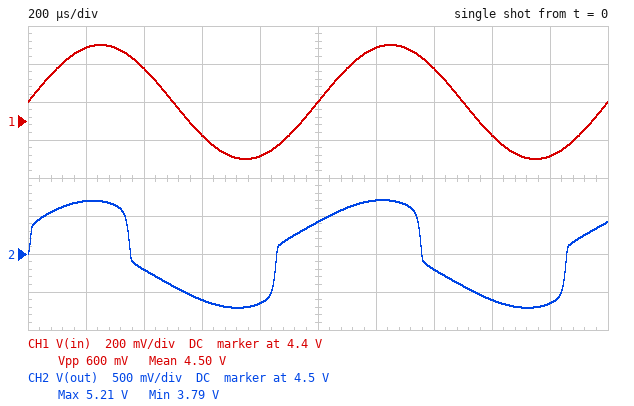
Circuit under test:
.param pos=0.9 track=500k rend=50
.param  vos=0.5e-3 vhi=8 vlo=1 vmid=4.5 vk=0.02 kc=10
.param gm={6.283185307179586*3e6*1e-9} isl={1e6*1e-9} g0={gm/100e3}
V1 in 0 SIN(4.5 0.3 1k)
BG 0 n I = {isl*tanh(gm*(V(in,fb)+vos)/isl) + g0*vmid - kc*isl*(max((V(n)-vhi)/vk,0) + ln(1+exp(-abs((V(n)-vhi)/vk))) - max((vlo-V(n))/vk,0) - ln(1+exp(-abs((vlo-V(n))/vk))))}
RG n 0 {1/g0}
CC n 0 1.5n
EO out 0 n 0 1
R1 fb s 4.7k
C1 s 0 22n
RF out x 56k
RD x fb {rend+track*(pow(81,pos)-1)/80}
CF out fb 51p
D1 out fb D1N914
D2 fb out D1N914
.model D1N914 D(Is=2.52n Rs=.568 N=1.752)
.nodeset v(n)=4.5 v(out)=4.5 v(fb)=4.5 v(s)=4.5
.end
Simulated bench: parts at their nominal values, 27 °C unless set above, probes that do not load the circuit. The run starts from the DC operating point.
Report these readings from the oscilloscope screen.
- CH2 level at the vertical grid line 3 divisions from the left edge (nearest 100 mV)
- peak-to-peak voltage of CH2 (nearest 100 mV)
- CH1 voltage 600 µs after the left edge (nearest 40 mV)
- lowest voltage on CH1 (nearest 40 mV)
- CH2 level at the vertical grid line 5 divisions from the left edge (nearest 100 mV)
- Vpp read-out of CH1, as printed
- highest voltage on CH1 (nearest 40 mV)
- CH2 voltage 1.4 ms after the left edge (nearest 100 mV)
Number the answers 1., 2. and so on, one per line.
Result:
1. 3.9 V
2. 1.4 V
3. 4.32 V
4. 4.20 V
5. 4.9 V
6. 600 mV
7. 4.80 V
8. 4.3 V
